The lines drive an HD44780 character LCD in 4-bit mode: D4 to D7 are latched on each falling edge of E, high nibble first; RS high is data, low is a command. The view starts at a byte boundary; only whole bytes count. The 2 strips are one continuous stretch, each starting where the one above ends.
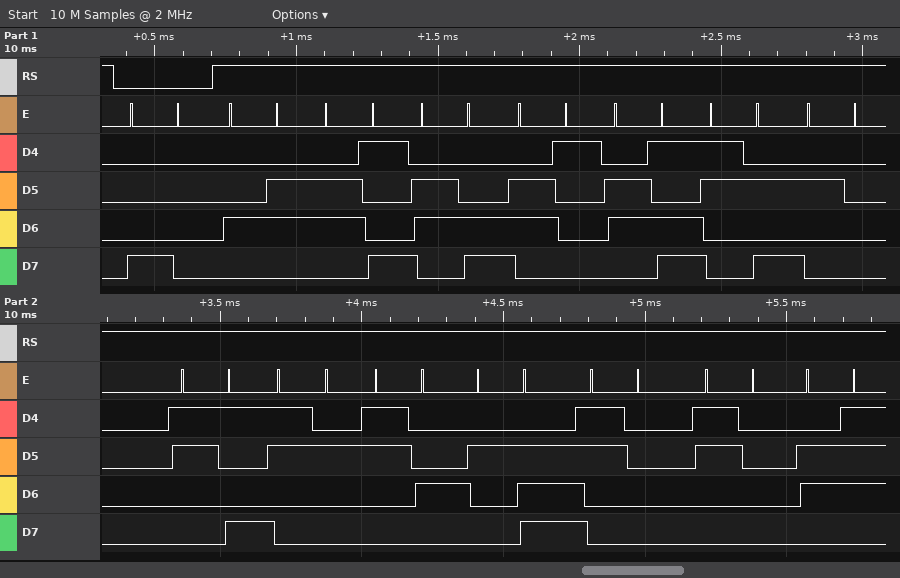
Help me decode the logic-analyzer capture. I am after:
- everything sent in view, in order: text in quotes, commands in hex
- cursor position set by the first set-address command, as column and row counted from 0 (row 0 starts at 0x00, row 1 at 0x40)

0x80 "Filam: 924.00g"
column 0, row 0
